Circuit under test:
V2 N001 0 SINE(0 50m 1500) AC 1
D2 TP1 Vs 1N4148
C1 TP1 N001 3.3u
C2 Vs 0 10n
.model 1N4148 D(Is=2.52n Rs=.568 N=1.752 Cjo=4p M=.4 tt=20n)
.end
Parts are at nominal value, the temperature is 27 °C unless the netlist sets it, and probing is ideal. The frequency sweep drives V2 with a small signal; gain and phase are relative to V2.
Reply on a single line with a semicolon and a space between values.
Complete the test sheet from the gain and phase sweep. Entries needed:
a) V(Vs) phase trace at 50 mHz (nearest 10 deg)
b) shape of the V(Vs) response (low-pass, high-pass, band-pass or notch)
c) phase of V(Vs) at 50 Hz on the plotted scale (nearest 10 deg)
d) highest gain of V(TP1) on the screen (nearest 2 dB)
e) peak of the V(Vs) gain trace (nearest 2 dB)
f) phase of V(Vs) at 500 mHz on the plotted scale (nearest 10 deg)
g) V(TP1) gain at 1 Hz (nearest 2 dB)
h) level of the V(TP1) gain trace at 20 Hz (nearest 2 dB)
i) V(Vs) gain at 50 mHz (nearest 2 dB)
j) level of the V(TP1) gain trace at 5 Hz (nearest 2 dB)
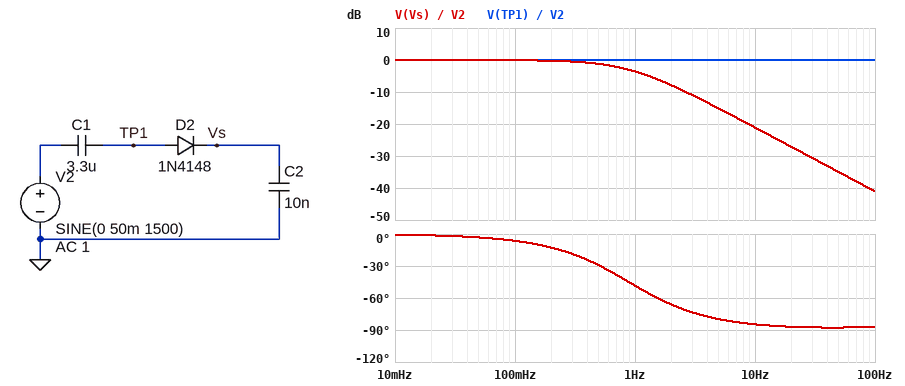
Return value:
0 deg; low-pass; -90 deg; 0 dB; 0 dB; -30 deg; 0 dB; 0 dB; 0 dB; 0 dB
